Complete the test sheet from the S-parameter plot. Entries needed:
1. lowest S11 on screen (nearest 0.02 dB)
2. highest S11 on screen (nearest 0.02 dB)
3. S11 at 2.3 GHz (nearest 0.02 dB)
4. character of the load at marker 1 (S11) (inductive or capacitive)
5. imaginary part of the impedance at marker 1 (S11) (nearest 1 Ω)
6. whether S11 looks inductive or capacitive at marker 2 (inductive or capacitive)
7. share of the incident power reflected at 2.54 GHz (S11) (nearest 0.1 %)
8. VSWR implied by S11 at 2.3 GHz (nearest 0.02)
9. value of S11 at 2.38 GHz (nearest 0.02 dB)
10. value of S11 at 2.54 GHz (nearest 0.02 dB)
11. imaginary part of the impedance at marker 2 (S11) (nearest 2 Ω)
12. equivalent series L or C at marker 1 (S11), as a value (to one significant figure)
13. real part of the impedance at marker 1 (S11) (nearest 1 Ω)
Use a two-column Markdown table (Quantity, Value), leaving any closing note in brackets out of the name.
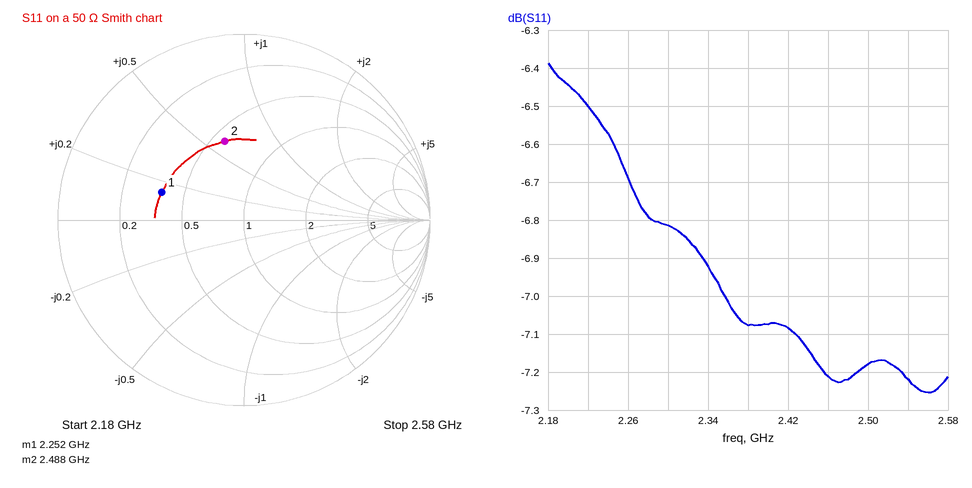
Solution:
| Quantity | Value |
|---|---|
| lowest S11 on screen | -7.26 dB |
| highest S11 on screen | -6.38 dB |
| S11 at 2.3 GHz | -6.82 dB |
| character of the load at marker 1 (S11) | inductive |
| imaginary part of the impedance at marker 1 (S11) | +7 Ω |
| whether S11 looks inductive or capacitive at marker 2 | inductive |
| share of the incident power reflected at 2.54 GHz (S11) | 19.0 % |
| VSWR implied by S11 at 2.3 GHz | 2.68 |
| value of S11 at 2.38 GHz | -7.08 dB |
| value of S11 at 2.54 GHz | -7.22 dB |
| imaginary part of the impedance at marker 2 (S11) | +30 Ω |
| equivalent series L or C at marker 1 (S11), as a value | 500 pH |
| real part of the impedance at marker 1 (S11) | 19 Ω |
